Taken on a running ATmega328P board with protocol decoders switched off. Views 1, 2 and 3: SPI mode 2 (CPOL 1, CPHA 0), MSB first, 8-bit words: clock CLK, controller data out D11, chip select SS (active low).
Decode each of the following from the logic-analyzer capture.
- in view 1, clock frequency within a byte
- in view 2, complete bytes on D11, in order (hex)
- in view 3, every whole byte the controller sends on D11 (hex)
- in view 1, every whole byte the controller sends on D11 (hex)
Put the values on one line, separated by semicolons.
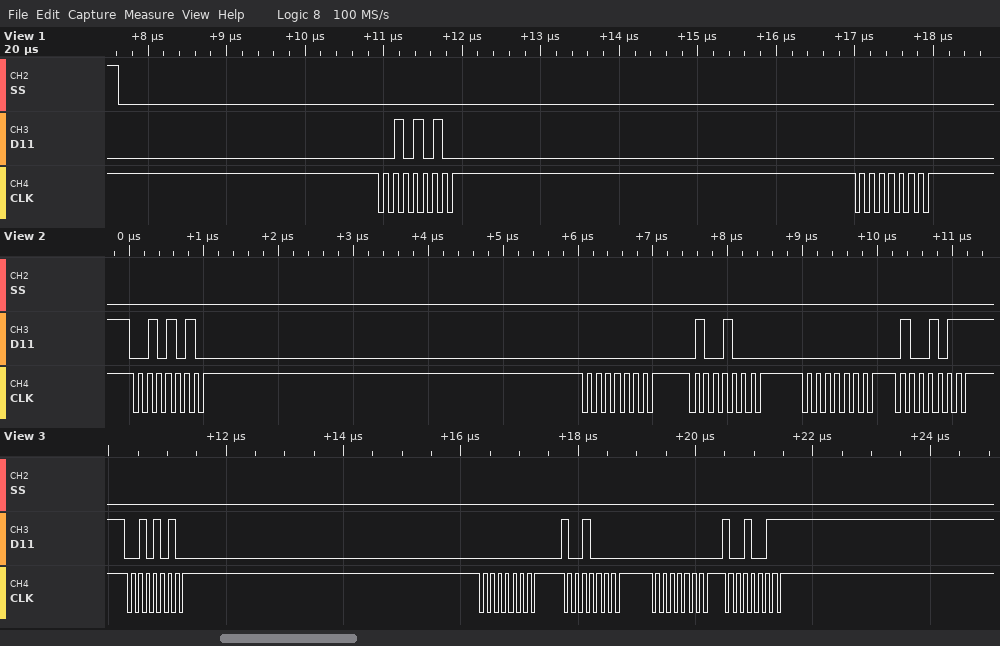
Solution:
8 MHz; 2A 00 48 00 4B; 2A 00 90 00 93; 2A 00
